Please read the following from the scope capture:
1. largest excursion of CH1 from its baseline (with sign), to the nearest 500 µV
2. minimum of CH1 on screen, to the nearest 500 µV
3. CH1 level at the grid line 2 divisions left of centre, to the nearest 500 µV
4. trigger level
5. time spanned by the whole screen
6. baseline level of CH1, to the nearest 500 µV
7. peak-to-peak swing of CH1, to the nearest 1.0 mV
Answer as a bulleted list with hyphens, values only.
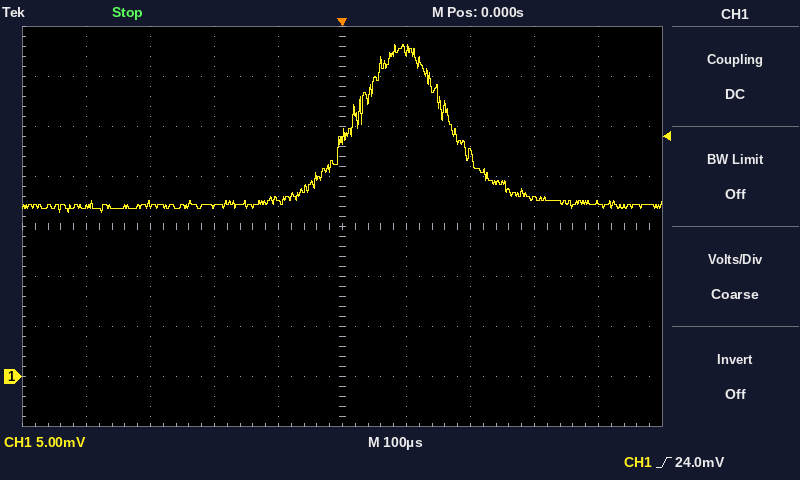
- +16.0 mV
- 16.5 mV
- 17.0 mV
- 24.0 mV
- 1 ms
- 17.0 mV
- 17.0 mV
